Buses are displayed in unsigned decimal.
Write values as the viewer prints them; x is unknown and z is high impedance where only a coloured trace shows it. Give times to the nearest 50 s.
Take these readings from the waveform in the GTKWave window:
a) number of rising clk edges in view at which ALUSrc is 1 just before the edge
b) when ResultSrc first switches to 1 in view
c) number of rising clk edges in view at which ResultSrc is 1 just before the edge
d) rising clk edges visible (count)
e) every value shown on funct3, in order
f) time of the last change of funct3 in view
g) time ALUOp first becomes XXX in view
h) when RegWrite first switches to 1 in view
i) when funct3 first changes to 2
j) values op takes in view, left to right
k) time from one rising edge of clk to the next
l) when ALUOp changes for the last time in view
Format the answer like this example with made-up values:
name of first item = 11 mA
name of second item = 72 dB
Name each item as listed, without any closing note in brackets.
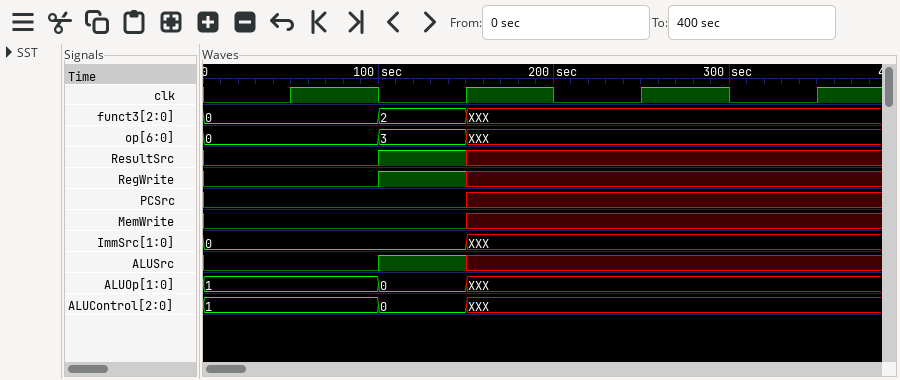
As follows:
number of rising clk edges in view at which ALUSrc is 1 just before the edge = 1
when ResultSrc first switches to 1 in view = 100 s
number of rising clk edges in view at which ResultSrc is 1 just before the edge = 1
rising clk edges visible = 4
every value shown on funct3, in order = 0, 2, XXX
time of the last change of funct3 in view = 150 s
time ALUOp first becomes XXX in view = 150 s
when RegWrite first switches to 1 in view = 100 s
when funct3 first changes to 2 = 100 s
values op takes in view, left to right = 0, 3, XXX
time from one rising edge of clk to the next = 100 s
when ALUOp changes for the last time in view = 150 s
